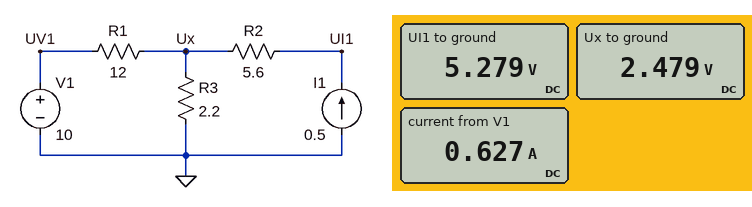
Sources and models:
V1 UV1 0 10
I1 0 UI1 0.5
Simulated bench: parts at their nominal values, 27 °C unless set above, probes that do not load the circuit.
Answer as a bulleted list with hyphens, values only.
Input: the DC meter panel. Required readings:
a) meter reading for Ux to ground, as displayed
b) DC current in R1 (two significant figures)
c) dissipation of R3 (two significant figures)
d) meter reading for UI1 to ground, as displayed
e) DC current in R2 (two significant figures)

- 2.479 V
- 630 mA
- 2.8 W
- 5.279 V
- 500 mA
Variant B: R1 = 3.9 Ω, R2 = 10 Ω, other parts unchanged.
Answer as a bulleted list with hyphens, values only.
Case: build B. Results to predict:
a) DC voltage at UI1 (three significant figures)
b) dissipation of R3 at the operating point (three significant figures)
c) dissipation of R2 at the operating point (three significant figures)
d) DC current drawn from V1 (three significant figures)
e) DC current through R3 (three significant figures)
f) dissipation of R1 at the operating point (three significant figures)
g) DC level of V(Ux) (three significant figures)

- 9.31 V
- 8.44 W
- 2.50 W
- 1.46 A
- 1.96 A
- 8.30 W
- 4.31 V
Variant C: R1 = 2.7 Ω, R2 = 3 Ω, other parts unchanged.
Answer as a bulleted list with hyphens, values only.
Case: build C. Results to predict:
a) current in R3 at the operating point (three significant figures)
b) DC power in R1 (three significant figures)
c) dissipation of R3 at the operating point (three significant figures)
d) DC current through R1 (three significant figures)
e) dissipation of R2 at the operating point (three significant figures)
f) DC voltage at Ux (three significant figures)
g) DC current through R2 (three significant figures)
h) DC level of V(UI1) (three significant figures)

- 2.32 A
- 8.91 W
- 11.8 W
- 1.82 A
- 750 mW
- 5.10 V
- 500 mA
- 6.60 V
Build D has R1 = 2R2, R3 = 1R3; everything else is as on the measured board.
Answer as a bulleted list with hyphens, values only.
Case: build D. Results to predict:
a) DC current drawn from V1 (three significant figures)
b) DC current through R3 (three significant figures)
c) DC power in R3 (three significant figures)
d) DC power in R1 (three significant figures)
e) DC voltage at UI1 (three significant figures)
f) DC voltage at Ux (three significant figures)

- 2.67 A
- 3.17 A
- 13.1 W
- 15.7 W
- 6.92 V
- 4.12 V
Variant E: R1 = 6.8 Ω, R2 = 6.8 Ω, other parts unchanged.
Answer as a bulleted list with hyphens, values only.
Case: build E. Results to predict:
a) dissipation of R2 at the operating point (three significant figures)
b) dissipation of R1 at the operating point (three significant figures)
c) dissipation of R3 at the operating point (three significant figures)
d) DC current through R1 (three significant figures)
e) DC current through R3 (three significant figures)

- 1.70 W
- 6.65 W
- 4.88 W
- 989 mA
- 1.49 A
